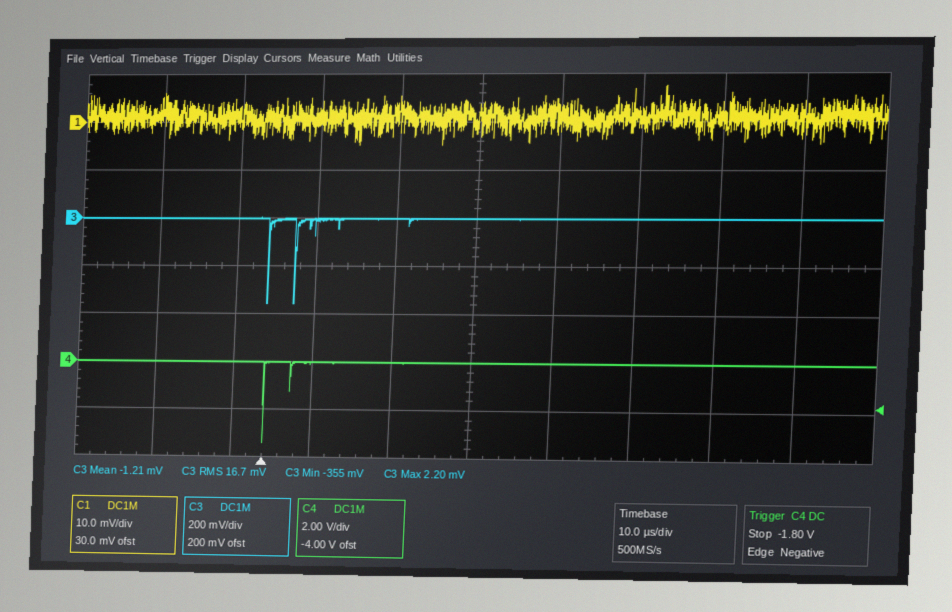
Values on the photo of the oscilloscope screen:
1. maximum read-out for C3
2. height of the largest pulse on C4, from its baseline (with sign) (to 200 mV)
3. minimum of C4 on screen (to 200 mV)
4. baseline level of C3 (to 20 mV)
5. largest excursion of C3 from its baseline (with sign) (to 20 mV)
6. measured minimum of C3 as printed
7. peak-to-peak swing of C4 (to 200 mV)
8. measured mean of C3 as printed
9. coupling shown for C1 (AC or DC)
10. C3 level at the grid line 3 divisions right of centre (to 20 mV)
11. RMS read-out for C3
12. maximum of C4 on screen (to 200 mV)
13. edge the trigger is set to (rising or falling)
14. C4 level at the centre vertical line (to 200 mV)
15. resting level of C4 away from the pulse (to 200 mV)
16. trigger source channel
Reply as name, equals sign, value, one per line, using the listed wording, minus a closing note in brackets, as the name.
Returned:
maximum read-out for C3 = 2.20 mV
height of the largest pulse on C4, from its baseline (with sign) = -3.4 V
minimum of C4 on screen = -3.4 V
baseline level of C3 = 0 mV
largest excursion of C3 from its baseline (with sign) = -360 mV
measured minimum of C3 as printed = -355 mV
peak-to-peak swing of C4 = 3.4 V
measured mean of C3 as printed = -1.21 mV
coupling shown for C1 = DC
C3 level at the grid line 3 divisions right of centre = 0 mV
RMS read-out for C3 = 16.7 mV
maximum of C4 on screen = 0.0 V
edge the trigger is set to = falling
C4 level at the centre vertical line = 0.0 V
resting level of C4 away from the pulse = 0.0 V
trigger source channel = C4
